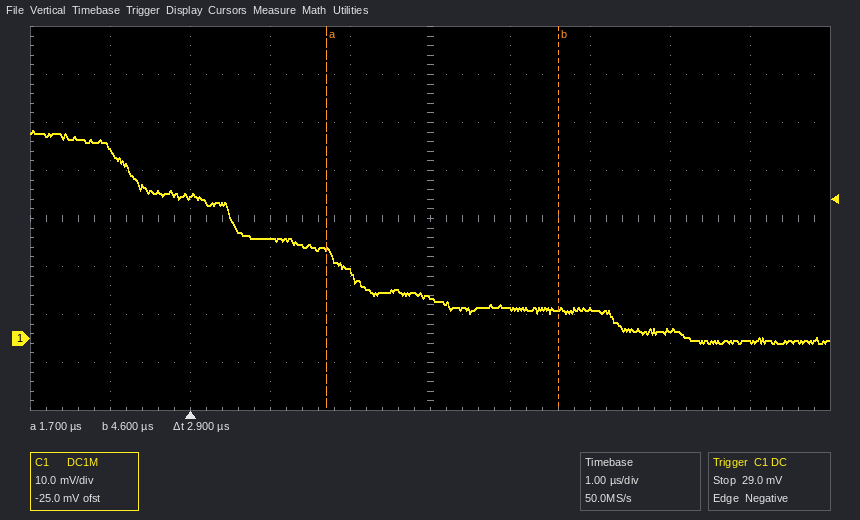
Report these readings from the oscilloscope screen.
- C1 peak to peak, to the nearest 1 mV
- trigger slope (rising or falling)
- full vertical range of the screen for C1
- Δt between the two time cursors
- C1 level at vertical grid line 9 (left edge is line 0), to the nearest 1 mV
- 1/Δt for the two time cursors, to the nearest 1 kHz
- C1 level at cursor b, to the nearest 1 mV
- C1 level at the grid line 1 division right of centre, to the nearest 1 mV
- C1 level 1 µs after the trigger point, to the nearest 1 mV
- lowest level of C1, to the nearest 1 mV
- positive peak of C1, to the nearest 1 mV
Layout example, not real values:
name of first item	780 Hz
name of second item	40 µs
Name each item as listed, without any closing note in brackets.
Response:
C1 peak to peak, to the nearest 1 mV	44 mV
trigger slope	falling
full vertical range of the screen for C1	80 mV
Δt between the two time cursors	2.9 µs
C1 level at vertical grid line 9 (left edge is line 0), to the nearest 1 mV	-1 mV
1/Δt for the two time cursors, to the nearest 1 kHz	345 kHz
C1 level at cursor b, to the nearest 1 mV	6 mV
C1 level at the grid line 1 division right of centre, to the nearest 1 mV	6 mV
C1 level 1 µs after the trigger point, to the nearest 1 mV	21 mV
lowest level of C1, to the nearest 1 mV	-1 mV
positive peak of C1, to the nearest 1 mV	43 mV
